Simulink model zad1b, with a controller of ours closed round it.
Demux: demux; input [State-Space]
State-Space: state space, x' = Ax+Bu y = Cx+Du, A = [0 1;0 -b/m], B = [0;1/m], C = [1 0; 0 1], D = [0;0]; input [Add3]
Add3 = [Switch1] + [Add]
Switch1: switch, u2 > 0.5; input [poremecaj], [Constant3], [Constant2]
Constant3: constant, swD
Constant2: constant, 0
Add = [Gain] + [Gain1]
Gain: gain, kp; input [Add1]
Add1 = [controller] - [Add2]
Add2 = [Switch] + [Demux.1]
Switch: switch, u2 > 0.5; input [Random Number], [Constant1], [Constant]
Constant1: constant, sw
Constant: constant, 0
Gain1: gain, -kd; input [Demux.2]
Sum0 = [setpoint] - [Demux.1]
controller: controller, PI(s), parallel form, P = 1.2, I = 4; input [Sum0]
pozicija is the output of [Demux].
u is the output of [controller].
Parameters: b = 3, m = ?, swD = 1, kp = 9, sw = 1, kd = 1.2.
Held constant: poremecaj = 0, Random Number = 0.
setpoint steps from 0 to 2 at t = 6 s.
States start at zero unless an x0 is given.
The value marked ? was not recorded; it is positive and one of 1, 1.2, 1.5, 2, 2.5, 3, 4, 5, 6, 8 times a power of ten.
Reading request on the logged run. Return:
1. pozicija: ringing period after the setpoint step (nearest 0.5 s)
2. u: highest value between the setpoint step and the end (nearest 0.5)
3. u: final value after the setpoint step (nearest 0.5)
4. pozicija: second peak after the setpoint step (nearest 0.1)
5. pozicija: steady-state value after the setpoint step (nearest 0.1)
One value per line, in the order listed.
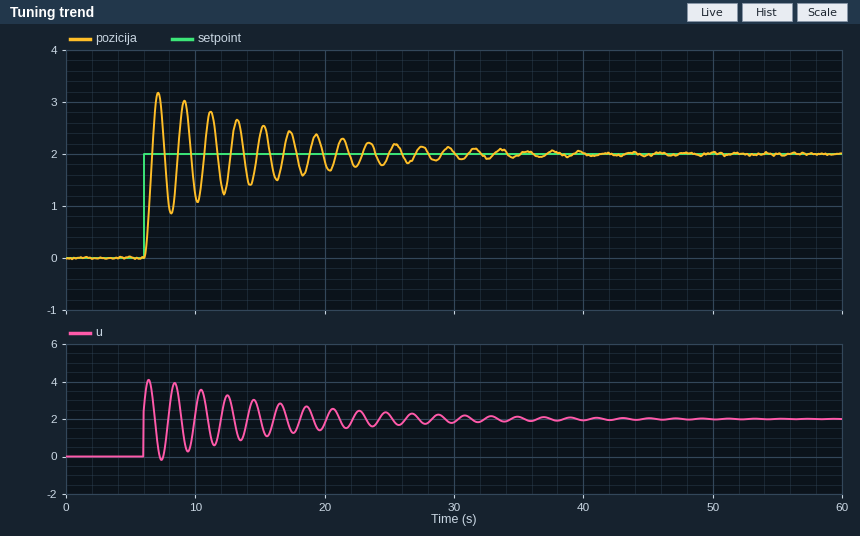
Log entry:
2.0 s
4.0
2.0
3.0
2.0
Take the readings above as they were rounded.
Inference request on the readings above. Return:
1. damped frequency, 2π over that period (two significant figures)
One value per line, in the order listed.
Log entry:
3.1 rad/s
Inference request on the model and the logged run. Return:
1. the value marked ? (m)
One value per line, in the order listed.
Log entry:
2
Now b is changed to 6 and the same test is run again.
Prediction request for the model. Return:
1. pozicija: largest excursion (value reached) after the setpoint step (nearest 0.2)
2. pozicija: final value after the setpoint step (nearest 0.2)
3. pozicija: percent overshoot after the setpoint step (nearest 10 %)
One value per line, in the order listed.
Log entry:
2.8
2.0
40 %
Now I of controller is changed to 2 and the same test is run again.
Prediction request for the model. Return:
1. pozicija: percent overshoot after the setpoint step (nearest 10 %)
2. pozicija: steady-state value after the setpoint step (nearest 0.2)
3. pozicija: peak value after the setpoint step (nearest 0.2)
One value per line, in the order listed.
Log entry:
20 %
2.0
2.4
